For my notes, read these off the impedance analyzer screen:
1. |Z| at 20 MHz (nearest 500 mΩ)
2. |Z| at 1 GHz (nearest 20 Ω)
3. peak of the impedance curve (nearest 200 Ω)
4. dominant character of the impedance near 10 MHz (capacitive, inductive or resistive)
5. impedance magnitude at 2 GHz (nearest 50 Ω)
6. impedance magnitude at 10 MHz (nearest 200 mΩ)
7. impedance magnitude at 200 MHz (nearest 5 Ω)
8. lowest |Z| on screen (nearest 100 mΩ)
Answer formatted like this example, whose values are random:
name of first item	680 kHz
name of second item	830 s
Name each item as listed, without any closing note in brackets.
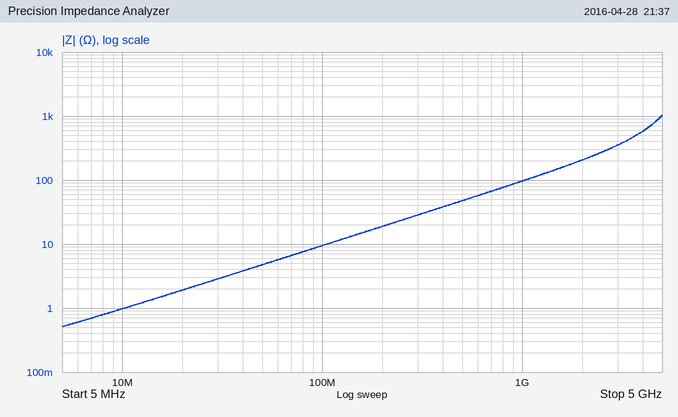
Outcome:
|Z| at 20 MHz	2.0 Ω
|Z| at 1 GHz	100 Ω
peak of the impedance curve	1.0 kΩ
dominant character of the impedance near 10 MHz	inductive
impedance magnitude at 2 GHz	200 Ω
impedance magnitude at 10 MHz	1.0 Ω
impedance magnitude at 200 MHz	20 Ω
lowest |Z| on screen	500 mΩ
